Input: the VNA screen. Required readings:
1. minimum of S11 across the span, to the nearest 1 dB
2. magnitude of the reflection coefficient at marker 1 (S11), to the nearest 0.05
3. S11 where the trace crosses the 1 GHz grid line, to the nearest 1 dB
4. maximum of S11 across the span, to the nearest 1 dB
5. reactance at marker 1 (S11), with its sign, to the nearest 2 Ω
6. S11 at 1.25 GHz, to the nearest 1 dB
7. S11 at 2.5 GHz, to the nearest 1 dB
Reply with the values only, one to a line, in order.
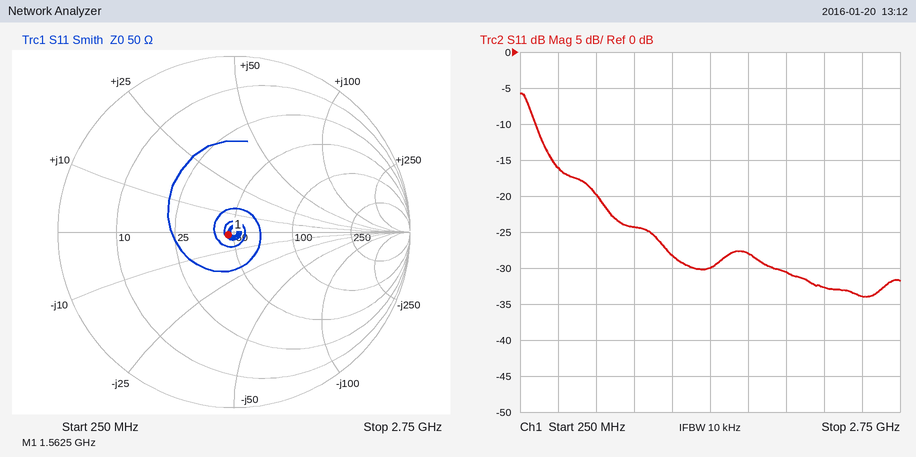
-34 dB
0.05
-24 dB
-6 dB
-2 Ω
-28 dB
-34 dB
